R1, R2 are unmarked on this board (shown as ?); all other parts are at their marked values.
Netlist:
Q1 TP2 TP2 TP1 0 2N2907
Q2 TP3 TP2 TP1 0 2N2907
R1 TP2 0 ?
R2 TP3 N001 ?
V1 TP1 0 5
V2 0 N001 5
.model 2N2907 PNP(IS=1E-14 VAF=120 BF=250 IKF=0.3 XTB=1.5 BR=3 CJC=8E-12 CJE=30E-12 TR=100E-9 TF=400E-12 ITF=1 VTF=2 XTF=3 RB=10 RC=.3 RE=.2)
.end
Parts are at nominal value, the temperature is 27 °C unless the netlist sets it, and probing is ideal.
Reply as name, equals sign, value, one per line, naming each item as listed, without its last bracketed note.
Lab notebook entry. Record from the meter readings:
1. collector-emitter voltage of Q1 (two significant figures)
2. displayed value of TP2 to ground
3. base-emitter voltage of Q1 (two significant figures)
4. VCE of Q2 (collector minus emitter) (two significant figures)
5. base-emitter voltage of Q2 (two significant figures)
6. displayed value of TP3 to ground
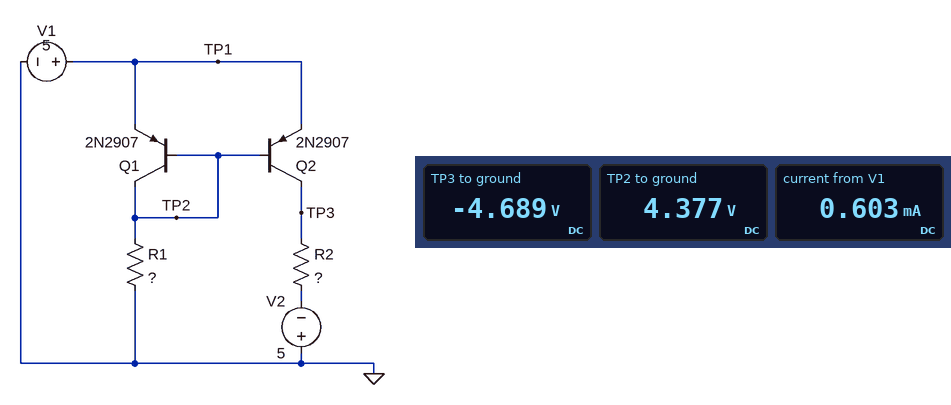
collector-emitter voltage of Q1 = -620 mV
displayed value of TP2 to ground = 4.377 V
base-emitter voltage of Q1 = -620 mV
VCE of Q2 (collector minus emitter) = -9.7 V
base-emitter voltage of Q2 = -620 mV
displayed value of TP3 to ground = -4.689 V
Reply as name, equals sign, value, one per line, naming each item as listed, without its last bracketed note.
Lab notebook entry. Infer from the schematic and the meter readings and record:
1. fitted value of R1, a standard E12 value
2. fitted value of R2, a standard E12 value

fitted value of R1, a standard E12 value = 15 kΩ
fitted value of R2, a standard E12 value = 1 kΩ
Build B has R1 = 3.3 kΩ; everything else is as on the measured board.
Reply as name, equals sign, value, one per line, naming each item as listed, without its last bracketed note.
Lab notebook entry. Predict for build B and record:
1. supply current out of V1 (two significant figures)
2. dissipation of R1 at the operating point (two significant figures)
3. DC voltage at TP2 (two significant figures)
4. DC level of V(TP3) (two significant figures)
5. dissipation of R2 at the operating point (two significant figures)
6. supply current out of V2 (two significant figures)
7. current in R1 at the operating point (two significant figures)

supply current out of V1 = 2.7 mA
dissipation of R1 at the operating point = 5.7 mW
DC voltage at TP2 = 4.3 V
DC level of V(TP3) = -3.6 V
dissipation of R2 at the operating point = 1.9 mW
supply current out of V2 = 1.4 mA
current in R1 at the operating point = 1.3 mA
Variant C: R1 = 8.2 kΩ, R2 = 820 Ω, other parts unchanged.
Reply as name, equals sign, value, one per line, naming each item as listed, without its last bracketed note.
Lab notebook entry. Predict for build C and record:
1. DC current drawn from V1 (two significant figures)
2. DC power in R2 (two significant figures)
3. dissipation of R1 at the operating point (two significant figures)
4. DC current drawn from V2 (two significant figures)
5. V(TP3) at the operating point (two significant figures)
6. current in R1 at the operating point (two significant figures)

DC current drawn from V1 = 1.1 mA
DC power in R2 = 260 µW
dissipation of R1 at the operating point = 2.3 mW
DC current drawn from V2 = 570 µA
V(TP3) at the operating point = -4.5 V
current in R1 at the operating point = 530 µA
